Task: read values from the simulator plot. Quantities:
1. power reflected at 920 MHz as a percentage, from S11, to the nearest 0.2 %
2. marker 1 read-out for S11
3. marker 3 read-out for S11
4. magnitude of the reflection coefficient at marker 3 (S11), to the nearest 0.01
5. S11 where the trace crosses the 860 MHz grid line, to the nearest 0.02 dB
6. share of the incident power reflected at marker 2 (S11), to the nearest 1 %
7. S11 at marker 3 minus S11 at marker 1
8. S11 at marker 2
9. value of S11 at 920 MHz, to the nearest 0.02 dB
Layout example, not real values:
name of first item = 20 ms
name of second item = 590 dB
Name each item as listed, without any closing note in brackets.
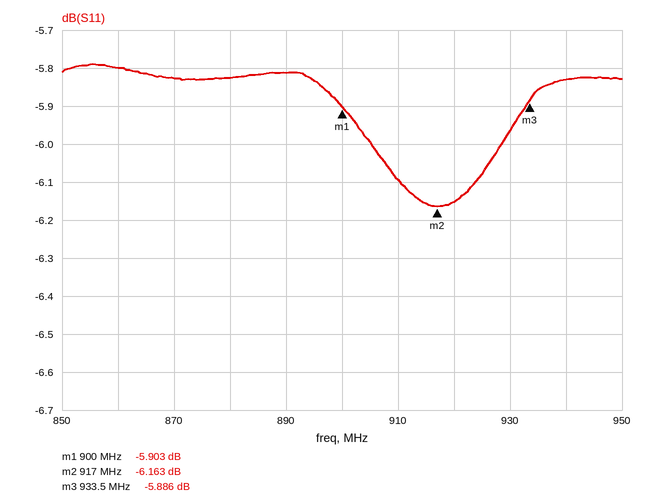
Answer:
power reflected at 920 MHz as a percentage, from S11, to the nearest 0.2 % = 24.2 %
marker 1 read-out for S11 = -5.903 dB
marker 3 read-out for S11 = -5.886 dB
magnitude of the reflection coefficient at marker 3 (S11), to the nearest 0.01 = 0.51
S11 where the trace crosses the 860 MHz grid line, to the nearest 0.02 dB = -5.80 dB
share of the incident power reflected at marker 2 (S11), to the nearest 1 % = 24 %
S11 at marker 3 minus S11 at marker 1 = 0.017 dB
S11 at marker 2 = -6.163 dB
value of S11 at 920 MHz, to the nearest 0.02 dB = -6.16 dB
